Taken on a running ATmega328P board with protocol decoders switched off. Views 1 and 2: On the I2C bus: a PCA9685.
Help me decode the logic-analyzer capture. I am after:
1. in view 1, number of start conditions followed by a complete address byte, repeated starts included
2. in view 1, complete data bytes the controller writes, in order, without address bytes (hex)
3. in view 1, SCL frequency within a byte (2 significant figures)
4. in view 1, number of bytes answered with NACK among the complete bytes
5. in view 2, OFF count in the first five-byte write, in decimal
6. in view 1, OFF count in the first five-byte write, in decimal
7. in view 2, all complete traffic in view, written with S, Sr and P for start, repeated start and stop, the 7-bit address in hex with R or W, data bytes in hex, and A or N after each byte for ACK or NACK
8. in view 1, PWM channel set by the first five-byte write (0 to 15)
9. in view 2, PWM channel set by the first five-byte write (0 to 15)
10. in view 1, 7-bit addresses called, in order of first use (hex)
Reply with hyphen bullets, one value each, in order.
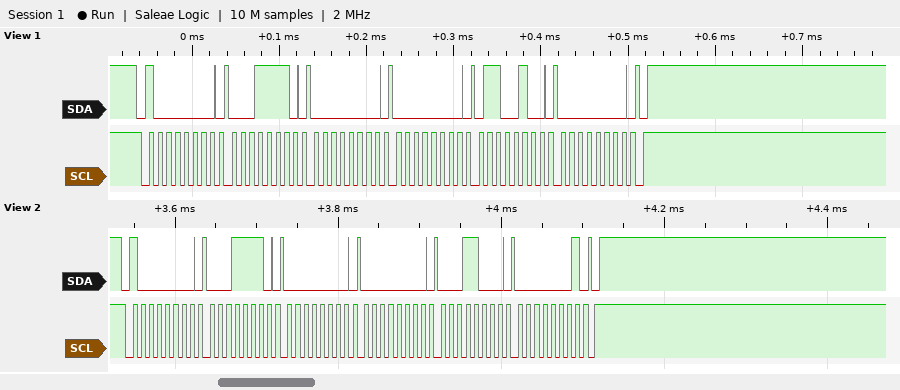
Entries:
- 1
- 1E 00 00 64 00
- 100 kHz
- 0
- 280
- 100
- S 40W A 1E A 00 A 00 A 18 A 01 A P
- 6
- 6
- 0x40
